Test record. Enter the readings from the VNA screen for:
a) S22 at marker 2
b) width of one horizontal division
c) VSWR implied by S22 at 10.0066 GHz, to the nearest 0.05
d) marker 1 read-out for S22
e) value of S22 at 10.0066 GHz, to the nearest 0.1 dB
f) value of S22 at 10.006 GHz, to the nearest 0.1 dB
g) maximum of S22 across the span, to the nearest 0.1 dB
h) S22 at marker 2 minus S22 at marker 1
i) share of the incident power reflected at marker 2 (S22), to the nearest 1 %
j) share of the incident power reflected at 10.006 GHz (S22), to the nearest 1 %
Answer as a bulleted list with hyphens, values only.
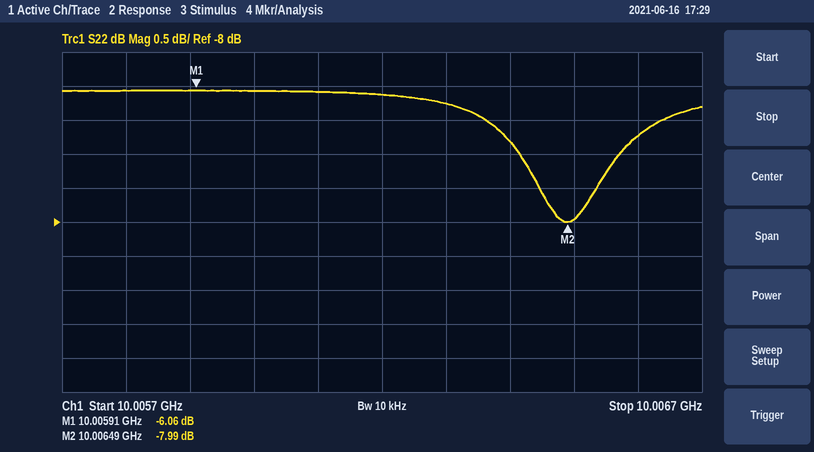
- -7.99 dB
- 100 kHz
- 2.70
- -6.06 dB
- -6.7 dB
- -6.1 dB
- -6.1 dB
- -1.93 dB
- 16 %
- 25 %
